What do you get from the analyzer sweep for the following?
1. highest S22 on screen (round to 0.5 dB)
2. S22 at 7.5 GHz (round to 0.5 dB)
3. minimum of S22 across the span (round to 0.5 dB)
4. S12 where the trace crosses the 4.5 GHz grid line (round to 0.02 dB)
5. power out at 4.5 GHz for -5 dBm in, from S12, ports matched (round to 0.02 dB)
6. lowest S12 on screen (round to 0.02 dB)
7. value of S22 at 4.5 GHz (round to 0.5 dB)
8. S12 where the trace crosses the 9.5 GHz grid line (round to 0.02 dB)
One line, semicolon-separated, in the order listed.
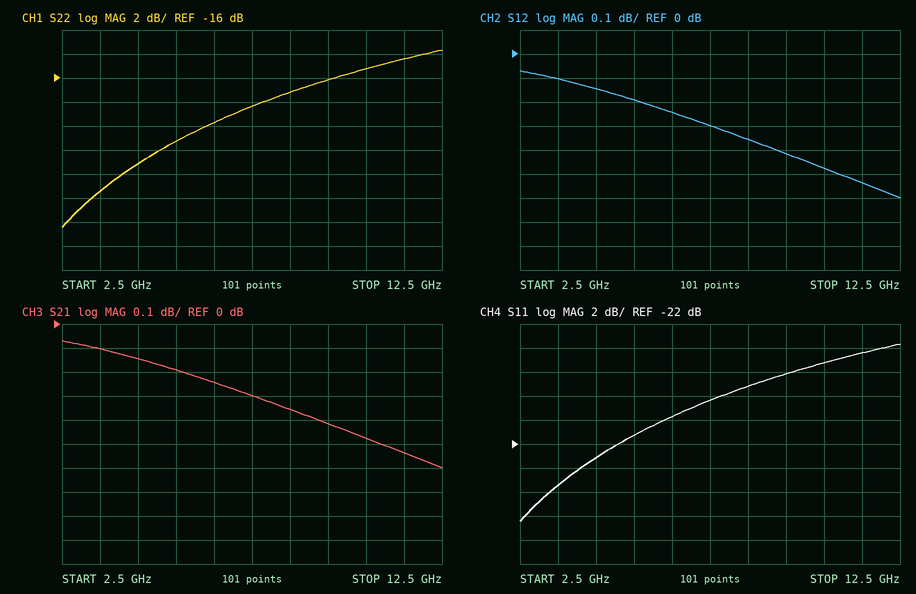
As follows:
-13.5 dB; -18.5 dB; -28.5 dB; -0.14 dB; -5.14 dBm; -0.60 dB; -23.0 dB; -0.42 dB
